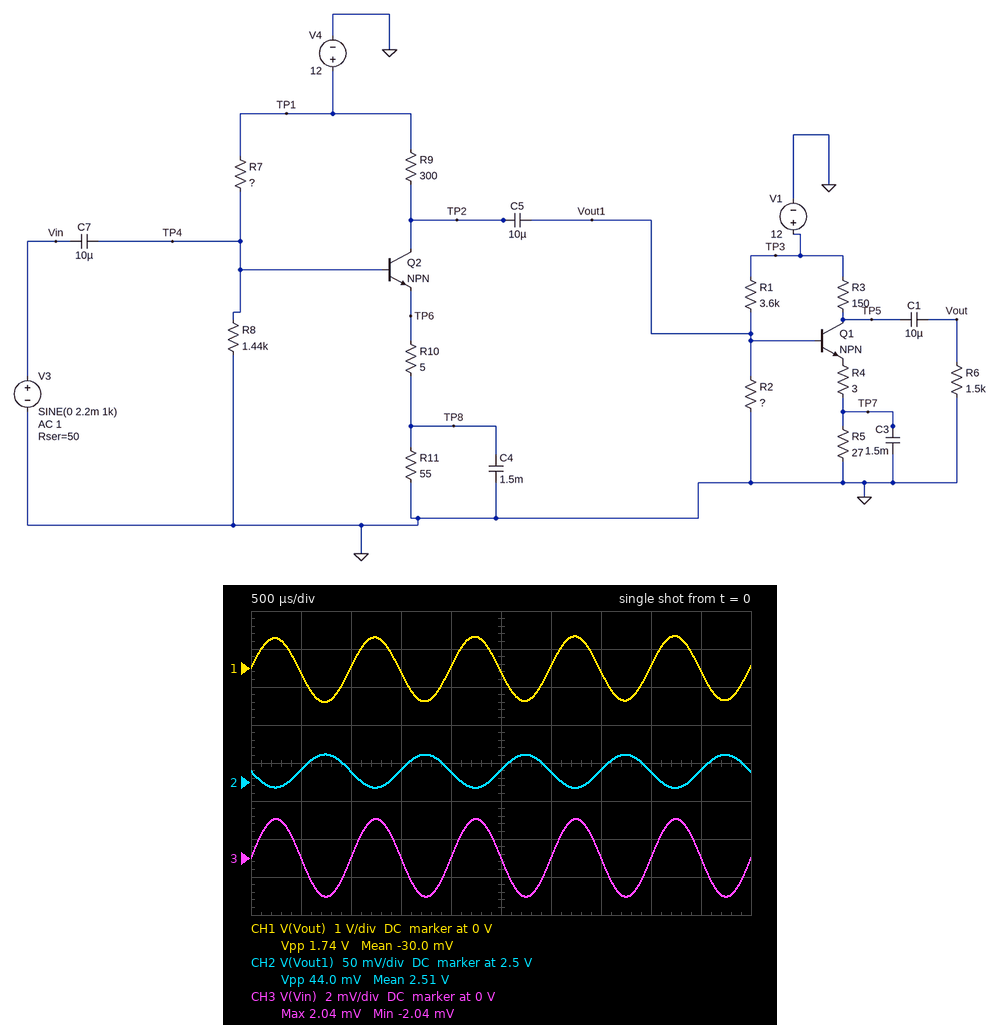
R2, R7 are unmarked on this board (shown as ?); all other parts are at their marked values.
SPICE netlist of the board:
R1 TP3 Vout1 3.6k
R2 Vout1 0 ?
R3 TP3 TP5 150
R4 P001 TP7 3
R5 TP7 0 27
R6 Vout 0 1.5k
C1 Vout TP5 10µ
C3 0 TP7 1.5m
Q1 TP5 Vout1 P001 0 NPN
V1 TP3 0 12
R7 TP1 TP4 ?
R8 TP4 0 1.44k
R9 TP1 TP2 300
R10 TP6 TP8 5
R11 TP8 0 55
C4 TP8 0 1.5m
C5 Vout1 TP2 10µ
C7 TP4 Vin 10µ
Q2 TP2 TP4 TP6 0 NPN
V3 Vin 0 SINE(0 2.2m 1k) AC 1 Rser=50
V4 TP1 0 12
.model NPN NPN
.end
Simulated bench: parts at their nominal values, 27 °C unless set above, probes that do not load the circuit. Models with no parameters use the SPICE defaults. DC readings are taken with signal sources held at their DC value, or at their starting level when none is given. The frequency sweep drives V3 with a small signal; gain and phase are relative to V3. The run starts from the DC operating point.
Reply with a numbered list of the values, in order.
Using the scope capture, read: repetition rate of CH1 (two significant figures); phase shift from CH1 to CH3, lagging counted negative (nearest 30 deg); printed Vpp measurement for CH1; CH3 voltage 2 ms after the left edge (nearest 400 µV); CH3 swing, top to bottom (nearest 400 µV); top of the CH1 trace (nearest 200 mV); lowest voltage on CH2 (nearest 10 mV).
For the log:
1. 1.0 kHz
2. 0 deg
3. 1.74 V
4. 0 V
5. 4.0 mV
6. 800 mV
7. 2.49 V
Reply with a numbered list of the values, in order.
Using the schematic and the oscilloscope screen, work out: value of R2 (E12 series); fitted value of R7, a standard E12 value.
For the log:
1. 1.2 kΩ
2. 15 kΩ
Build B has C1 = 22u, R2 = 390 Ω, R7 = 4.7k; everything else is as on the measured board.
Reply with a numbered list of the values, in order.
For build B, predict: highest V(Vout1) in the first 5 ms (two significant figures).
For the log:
1. 1.2 V
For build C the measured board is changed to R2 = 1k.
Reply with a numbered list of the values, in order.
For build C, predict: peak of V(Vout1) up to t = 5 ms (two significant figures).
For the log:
1. 2.3 V
